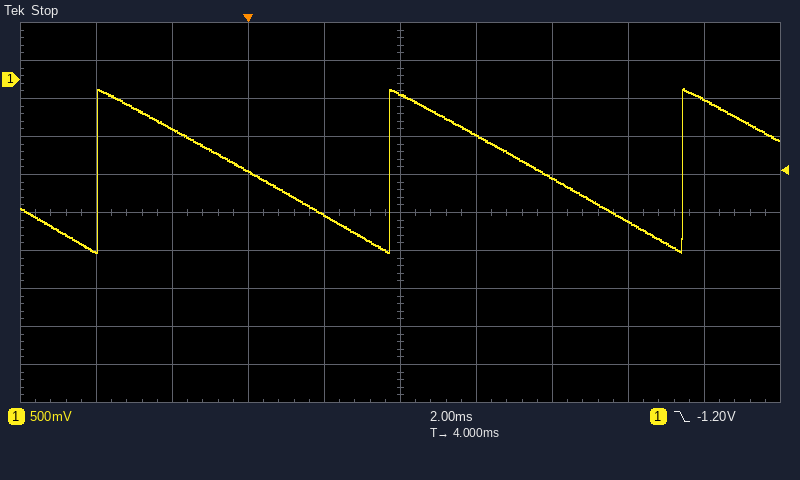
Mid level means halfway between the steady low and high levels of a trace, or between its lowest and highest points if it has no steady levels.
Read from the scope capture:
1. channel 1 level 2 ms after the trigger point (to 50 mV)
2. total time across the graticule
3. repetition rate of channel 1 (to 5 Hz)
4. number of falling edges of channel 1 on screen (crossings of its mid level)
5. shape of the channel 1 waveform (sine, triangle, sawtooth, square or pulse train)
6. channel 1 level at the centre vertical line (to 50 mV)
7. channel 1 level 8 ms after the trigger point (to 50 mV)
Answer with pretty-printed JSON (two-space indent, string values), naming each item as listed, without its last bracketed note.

{
  "channel 1 level 2 ms after the trigger point": "-1.80 V",
  "total time across the graticule": "20 ms",
  "repetition rate of channel 1": "130 Hz",
  "number of falling edges of channel 1 on screen": "2",
  "shape of the channel 1 waveform": "sawtooth",
  "channel 1 level at the centre vertical line": "-200 mV",
  "channel 1 level 8 ms after the trigger point": "-1.30 V"
}
